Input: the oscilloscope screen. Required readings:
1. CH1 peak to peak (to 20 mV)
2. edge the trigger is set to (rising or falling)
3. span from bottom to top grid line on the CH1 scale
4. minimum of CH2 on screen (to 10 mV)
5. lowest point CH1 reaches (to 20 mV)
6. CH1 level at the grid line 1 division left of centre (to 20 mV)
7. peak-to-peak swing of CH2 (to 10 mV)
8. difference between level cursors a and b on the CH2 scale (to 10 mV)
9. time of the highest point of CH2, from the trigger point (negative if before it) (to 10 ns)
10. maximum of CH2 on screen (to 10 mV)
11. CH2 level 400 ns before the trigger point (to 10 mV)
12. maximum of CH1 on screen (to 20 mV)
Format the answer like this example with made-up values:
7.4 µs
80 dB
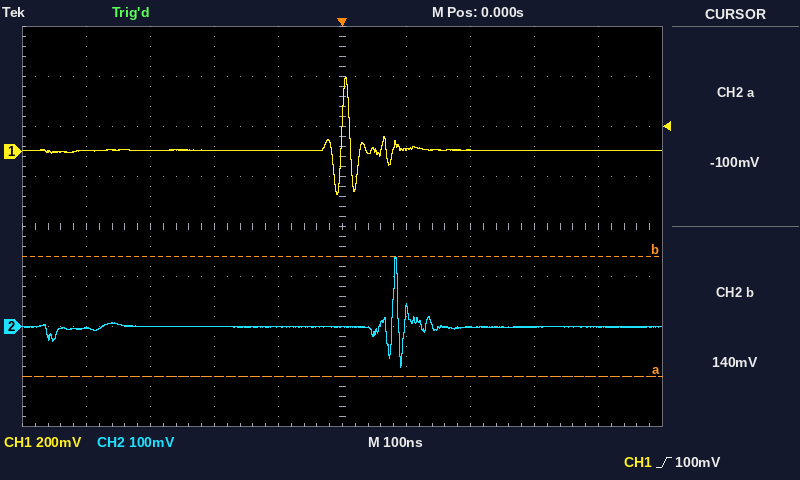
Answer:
480 mV
rising
1.6 V
-80 mV
-180 mV
0 mV
220 mV
240 mV
+80 ns
140 mV
0 mV
300 mV
